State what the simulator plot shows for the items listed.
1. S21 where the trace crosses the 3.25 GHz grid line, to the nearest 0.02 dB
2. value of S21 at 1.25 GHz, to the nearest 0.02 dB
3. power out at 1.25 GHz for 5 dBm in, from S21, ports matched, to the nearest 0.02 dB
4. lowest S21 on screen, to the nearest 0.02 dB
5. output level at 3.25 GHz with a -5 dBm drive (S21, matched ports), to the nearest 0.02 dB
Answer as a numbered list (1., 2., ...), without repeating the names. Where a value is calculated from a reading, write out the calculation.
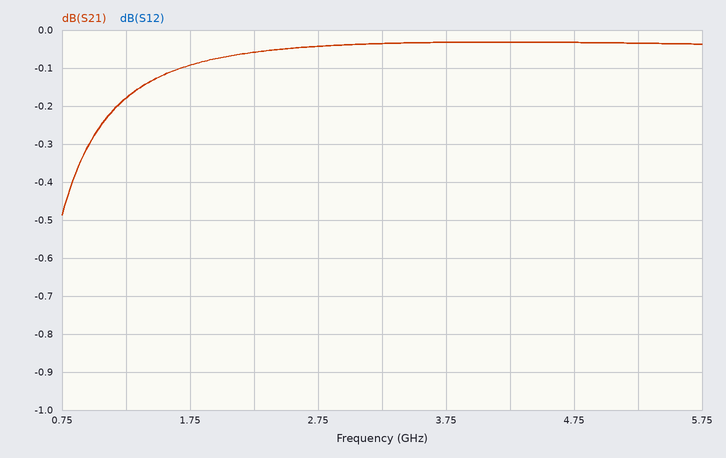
1. -0.04 dB
2. -0.18 dB
3. 5 dBm + (-0.18 dB) = 4.82 dBm
4. -0.48 dB
5. -5 dBm + (-0.04 dB) = -5.04 dBm
